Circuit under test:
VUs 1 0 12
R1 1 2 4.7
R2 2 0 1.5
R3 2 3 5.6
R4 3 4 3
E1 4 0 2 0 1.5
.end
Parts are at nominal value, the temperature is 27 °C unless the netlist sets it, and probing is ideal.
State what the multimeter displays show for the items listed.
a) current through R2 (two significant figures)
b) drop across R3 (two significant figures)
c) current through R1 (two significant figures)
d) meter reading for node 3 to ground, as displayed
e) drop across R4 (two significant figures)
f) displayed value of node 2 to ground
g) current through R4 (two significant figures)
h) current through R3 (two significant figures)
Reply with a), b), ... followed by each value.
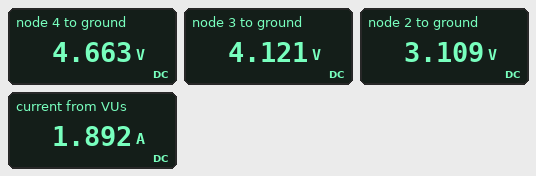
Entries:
a) 2.1 A
b) 1.0 V
c) 1.9 A
d) 4.121 V
e) 540 mV
f) 3.109 V
g) 180 mA
h) 180 mA
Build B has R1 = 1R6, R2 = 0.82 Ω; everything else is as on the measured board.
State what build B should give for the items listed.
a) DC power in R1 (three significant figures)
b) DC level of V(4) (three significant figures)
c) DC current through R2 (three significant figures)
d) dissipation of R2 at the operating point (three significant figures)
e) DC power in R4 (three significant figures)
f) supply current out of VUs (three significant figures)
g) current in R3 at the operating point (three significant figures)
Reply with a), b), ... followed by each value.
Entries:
a) 38.0 W
b) 6.30 V
c) 5.12 A
d) 21.5 W
e) 179 mW
f) 4.88 A
g) 244 mA
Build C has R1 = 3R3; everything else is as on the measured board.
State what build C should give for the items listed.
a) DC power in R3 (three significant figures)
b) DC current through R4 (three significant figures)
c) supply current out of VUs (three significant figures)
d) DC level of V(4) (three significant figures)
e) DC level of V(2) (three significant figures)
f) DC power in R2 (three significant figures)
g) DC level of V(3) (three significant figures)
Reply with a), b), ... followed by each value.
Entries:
a) 301 mW
b) 232 mA
c) 2.43 A
d) 5.98 V
e) 3.99 V
f) 10.6 W
g) 5.29 V
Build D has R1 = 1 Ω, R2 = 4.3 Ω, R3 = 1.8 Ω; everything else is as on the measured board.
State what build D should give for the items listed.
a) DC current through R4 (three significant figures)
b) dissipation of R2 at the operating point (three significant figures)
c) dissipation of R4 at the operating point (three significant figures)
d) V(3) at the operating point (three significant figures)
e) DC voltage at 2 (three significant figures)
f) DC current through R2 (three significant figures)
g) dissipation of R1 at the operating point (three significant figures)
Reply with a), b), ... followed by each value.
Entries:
a) 1.11 A
b) 26.3 W
c) 3.68 W
d) 12.6 V
e) 10.6 V
f) 2.47 A
g) 1.86 W
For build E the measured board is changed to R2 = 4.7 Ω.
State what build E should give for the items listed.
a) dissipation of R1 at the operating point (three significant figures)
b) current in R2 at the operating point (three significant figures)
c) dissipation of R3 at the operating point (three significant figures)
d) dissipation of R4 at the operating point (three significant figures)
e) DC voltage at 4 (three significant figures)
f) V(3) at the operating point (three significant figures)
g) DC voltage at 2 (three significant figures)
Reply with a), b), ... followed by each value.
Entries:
a) 5.43 W
b) 1.48 A
c) 914 mW
d) 490 mW
e) 10.4 V
f) 9.21 V
g) 6.95 V
